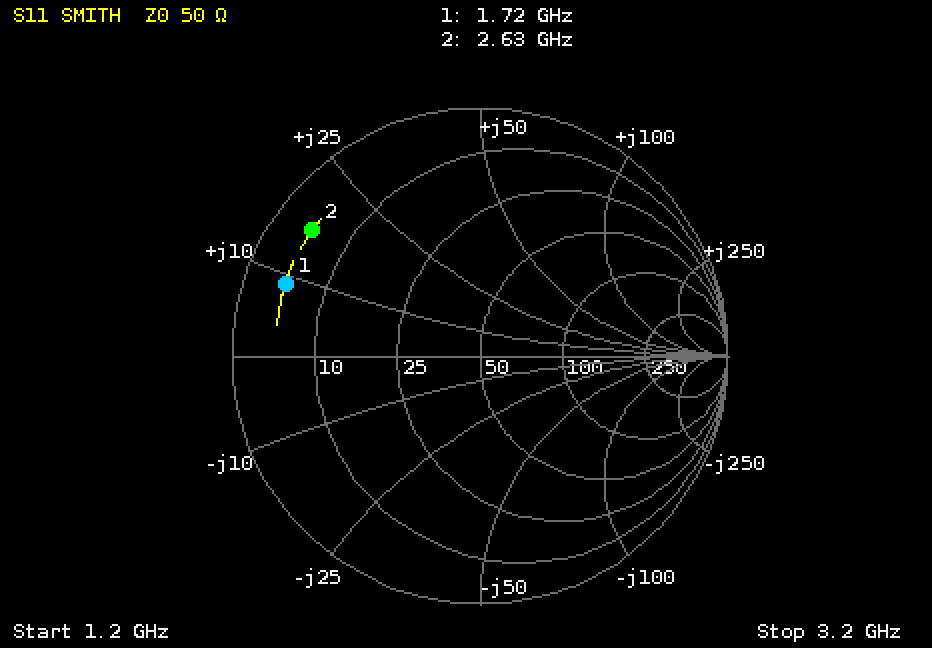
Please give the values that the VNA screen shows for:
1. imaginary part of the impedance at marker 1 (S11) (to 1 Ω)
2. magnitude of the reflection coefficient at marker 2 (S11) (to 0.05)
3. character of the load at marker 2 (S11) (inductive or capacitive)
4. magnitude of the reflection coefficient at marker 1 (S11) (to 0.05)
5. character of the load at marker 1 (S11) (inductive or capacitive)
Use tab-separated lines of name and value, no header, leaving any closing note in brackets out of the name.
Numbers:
imaginary part of the impedance at marker 1 (S11)	+9 Ω
magnitude of the reflection coefficient at marker 2 (S11)	0.85
character of the load at marker 2 (S11)	inductive
magnitude of the reflection coefficient at marker 1 (S11)	0.85
character of the load at marker 1 (S11)	inductive
